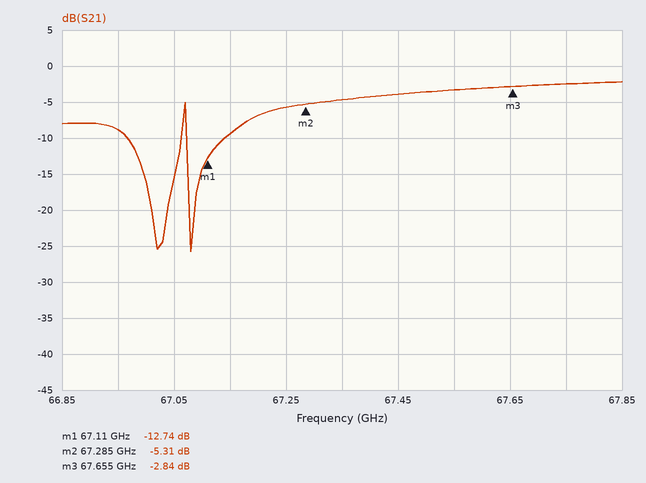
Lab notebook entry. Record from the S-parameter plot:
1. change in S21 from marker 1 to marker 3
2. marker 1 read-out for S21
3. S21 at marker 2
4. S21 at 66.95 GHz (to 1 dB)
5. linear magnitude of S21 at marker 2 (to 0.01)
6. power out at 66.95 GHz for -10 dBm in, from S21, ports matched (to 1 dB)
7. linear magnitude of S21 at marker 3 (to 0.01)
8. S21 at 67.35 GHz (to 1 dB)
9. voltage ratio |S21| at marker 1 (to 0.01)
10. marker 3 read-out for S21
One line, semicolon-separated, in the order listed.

9.90 dB; -12.74 dB; -5.31 dB; -9 dB; 0.54; -19 dBm; 0.72; -5 dB; 0.23; -2.84 dB
